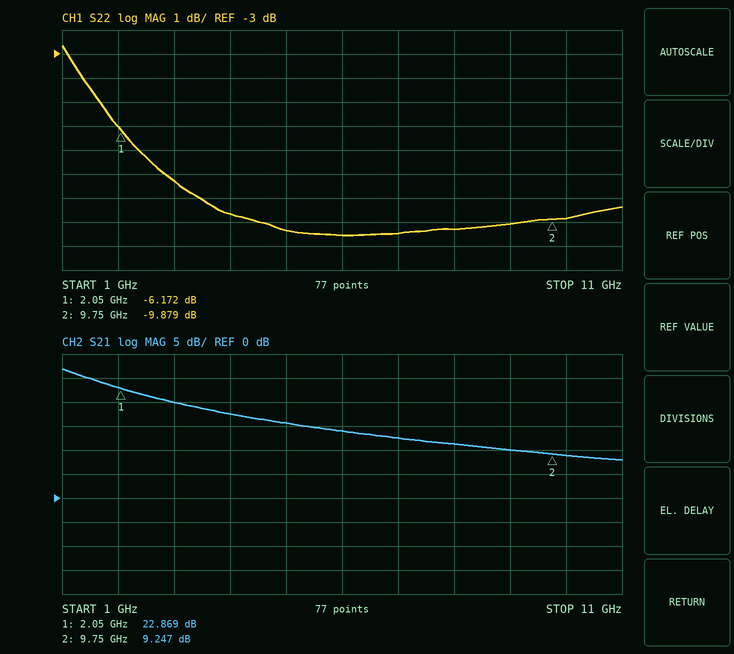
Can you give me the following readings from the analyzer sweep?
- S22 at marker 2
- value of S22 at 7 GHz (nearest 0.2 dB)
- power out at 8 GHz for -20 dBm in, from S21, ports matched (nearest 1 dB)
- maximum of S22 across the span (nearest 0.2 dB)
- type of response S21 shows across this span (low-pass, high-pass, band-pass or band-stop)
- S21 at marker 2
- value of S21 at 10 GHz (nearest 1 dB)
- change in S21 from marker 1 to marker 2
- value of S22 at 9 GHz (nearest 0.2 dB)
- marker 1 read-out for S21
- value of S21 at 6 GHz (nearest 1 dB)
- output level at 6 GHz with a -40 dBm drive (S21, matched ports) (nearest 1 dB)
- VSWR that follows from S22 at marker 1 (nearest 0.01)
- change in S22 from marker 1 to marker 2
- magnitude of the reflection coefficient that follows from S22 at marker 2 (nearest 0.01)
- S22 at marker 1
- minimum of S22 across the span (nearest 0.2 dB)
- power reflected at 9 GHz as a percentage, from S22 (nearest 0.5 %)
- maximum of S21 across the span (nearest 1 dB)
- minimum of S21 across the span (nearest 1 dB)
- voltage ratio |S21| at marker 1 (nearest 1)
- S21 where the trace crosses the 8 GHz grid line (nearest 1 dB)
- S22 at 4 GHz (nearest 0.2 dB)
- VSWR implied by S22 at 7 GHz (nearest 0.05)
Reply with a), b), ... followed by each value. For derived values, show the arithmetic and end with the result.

a) -9.879 dB
b) -10.4 dB
c) -20 dBm + (11 dB) = -9 dBm
d) -2.6 dB
e) low-pass
f) 9.247 dB
g) 9 dB
h) 9.247 − (22.869) = -13.622 dB
i) -10.0 dB
j) 22.869 dB
k) 14 dB
l) -40 dBm + (14 dB) = -26 dBm
m) (1 + 0.4914)/(1 − 0.4914) ≈ 2.93
n) -9.879 − (-6.172) = -3.707 dB
o) 10^(-9.879/20) ≈ 0.32
p) -6.172 dB
q) -10.6 dB
r) 10^(-10/10) ≈ 10.0 %
s) 27 dB
t) 8 dB
u) 10^(22.869/20) ≈ 14
v) 11 dB
w) -9.6 dB
x) |Γ| = 10^(-10.4/20) = 0.3020; VSWR = (1 + 0.3020)/(1 − 0.3020) ≈ 1.87, so 1.85 to the nearest 0.05
